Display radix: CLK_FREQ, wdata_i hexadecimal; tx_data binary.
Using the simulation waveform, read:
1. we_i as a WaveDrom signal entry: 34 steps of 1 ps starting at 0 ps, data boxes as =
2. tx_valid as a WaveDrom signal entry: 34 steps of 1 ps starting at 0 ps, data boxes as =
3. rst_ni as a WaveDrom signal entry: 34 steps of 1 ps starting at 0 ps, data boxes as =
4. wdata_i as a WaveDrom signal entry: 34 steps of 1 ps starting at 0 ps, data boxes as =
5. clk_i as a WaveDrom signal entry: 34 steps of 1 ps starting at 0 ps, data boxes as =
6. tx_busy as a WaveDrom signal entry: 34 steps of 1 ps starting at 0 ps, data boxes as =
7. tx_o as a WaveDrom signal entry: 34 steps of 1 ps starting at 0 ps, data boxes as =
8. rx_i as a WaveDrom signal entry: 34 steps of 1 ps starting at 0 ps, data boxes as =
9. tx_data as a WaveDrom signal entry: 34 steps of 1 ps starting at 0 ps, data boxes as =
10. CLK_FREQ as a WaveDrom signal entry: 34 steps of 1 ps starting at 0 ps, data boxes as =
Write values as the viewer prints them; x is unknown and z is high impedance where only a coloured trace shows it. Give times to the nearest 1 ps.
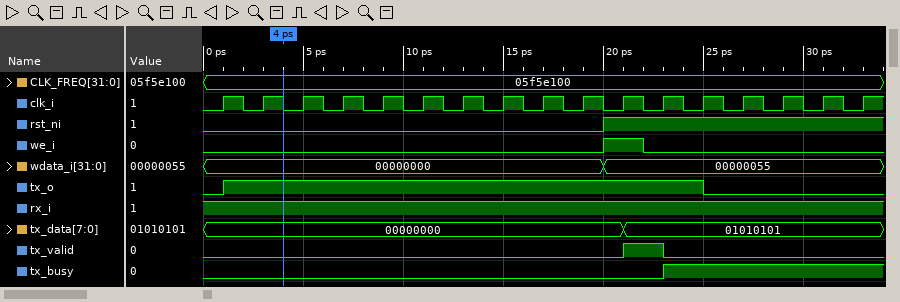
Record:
{name: 'we_i', wave: '0...................1.0...........'}
{name: 'tx_valid', wave: '0....................1.0..........'}
{name: 'rst_ni', wave: '0...................1.............'}
{name: 'wdata_i', wave: '=...................=.............', data: '00000000 00000055'}
{name: 'clk_i', wave: '0101010101010101010101010101010101'}
{name: 'tx_busy', wave: '0......................1..........'}
{name: 'tx_o', wave: '01.......................0........'}
{name: 'rx_i', wave: '1.................................'}
{name: 'tx_data', wave: '=....................=............', data: '00000000 01010101'}
{name: 'CLK_FREQ', wave: '=.................................', data: '05f5e100'}
